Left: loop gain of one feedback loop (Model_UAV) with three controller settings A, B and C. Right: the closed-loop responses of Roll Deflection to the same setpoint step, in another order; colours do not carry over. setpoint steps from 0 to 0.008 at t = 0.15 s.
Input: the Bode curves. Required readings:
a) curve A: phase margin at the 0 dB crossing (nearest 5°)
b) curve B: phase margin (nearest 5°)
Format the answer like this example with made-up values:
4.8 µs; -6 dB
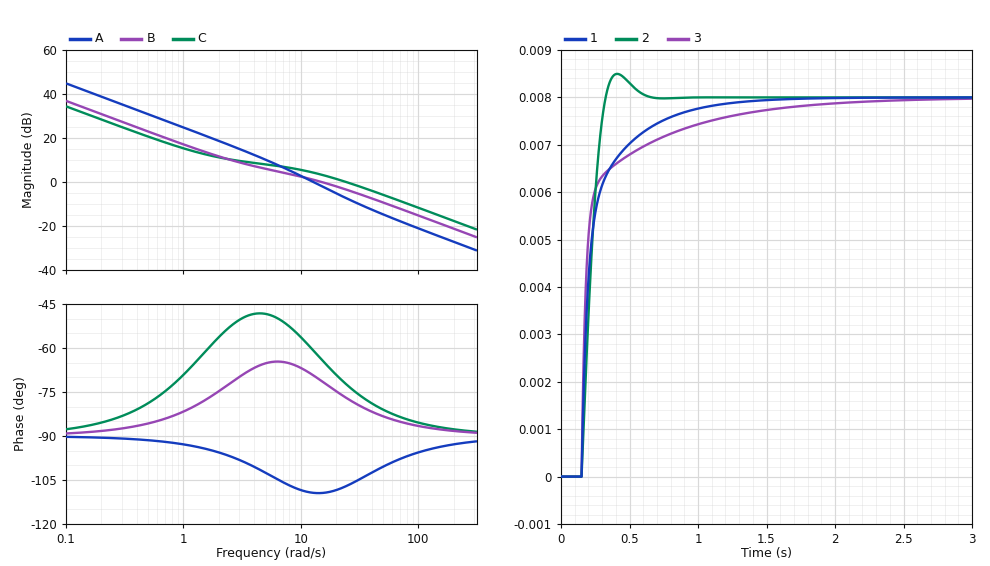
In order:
70°; 110°
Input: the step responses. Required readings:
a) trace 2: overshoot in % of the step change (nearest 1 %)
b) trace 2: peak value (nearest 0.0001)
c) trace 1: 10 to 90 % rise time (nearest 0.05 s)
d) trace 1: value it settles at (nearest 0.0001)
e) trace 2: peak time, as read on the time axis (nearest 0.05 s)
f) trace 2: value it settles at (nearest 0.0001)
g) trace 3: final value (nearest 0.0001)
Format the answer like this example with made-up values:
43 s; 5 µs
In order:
6 %; 0.0085; 0.40 s; 0.0080; 0.40 s; 0.0080; 0.0080
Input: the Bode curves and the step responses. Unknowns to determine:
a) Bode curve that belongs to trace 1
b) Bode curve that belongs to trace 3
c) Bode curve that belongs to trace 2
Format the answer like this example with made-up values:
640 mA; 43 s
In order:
B; C; A
